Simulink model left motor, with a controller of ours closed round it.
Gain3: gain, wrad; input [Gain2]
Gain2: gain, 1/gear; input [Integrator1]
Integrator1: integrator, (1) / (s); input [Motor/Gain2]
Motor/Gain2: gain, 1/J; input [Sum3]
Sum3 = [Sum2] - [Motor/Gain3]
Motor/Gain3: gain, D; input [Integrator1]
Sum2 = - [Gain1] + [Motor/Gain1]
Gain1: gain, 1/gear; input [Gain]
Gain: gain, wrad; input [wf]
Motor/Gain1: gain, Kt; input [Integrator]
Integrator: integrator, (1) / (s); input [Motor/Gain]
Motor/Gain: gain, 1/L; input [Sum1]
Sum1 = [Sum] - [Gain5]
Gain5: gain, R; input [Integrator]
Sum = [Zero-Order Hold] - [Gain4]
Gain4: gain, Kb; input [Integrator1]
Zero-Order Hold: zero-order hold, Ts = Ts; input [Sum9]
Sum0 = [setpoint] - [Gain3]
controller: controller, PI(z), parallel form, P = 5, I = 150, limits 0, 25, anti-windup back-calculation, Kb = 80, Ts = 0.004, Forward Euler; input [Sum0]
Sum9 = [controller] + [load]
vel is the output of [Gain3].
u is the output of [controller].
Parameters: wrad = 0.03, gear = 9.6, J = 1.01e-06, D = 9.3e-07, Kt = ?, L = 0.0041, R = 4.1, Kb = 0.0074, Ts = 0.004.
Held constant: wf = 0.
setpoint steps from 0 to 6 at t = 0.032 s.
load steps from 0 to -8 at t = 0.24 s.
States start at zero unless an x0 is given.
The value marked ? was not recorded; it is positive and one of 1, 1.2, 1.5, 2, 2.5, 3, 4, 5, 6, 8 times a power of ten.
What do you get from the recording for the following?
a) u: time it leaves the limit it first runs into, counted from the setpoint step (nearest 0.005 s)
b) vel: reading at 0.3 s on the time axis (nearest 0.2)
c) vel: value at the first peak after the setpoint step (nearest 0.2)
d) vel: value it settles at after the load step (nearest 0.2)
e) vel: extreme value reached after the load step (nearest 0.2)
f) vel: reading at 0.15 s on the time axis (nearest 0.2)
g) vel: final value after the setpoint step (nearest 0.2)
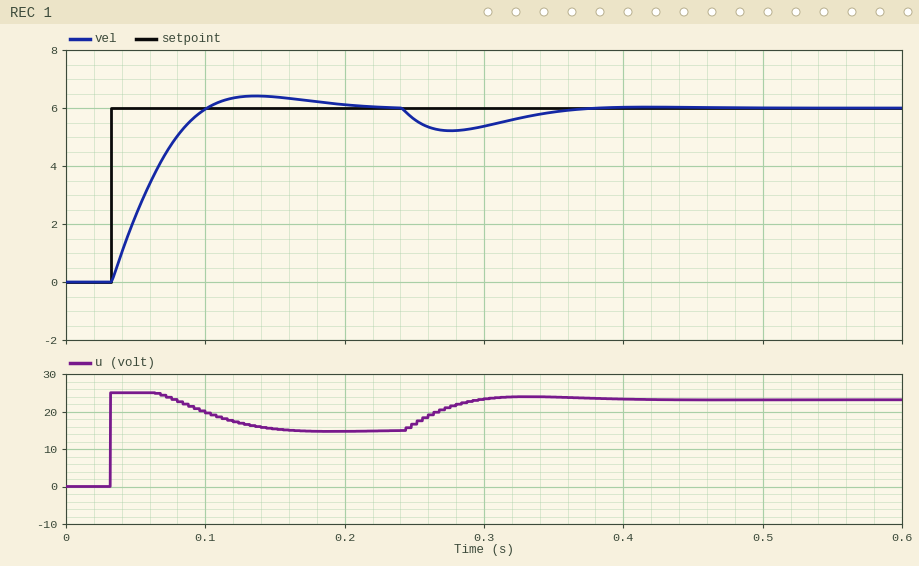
0.035 s
5.4
6.4
6.0
5.2
6.4
6.0
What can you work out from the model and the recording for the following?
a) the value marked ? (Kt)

0.008
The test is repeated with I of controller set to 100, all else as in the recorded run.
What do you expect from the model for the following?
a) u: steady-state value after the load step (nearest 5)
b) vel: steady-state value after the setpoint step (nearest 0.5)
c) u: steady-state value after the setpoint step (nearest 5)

25
6.0
15
